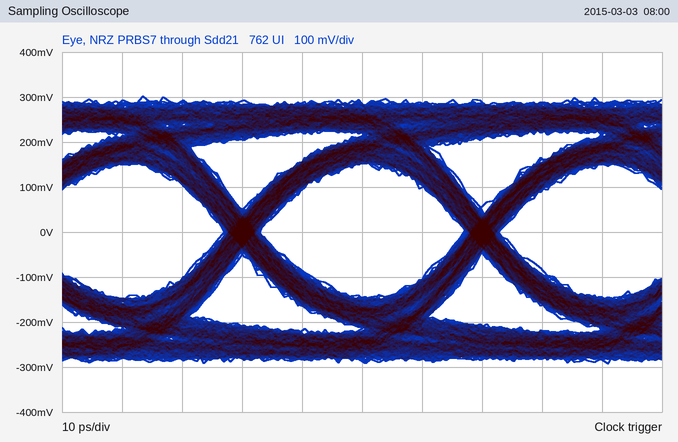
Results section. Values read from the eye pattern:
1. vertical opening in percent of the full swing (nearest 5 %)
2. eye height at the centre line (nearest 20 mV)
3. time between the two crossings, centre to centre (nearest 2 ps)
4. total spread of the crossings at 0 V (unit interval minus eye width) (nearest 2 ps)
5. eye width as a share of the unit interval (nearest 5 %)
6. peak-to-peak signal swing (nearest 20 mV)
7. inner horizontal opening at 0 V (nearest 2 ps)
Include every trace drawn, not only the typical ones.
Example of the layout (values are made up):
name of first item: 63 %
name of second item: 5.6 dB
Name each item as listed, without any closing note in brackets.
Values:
vertical opening in percent of the full swing: 50 %
eye height at the centre line: 300 mV
time between the two crossings, centre to centre: 40 ps
total spread of the crossings at 0 V (unit interval minus eye width): 6 ps
eye width as a share of the unit interval: 85 %
peak-to-peak signal swing: 600 mV
inner horizontal opening at 0 V: 34 ps
